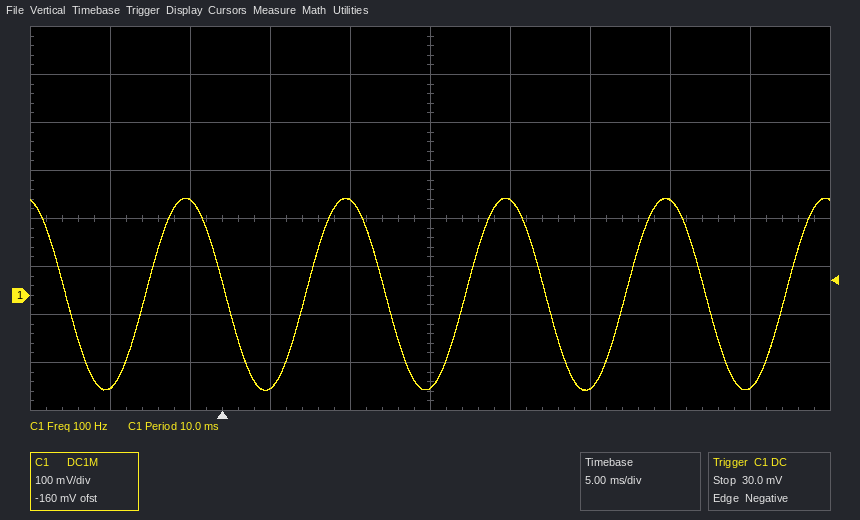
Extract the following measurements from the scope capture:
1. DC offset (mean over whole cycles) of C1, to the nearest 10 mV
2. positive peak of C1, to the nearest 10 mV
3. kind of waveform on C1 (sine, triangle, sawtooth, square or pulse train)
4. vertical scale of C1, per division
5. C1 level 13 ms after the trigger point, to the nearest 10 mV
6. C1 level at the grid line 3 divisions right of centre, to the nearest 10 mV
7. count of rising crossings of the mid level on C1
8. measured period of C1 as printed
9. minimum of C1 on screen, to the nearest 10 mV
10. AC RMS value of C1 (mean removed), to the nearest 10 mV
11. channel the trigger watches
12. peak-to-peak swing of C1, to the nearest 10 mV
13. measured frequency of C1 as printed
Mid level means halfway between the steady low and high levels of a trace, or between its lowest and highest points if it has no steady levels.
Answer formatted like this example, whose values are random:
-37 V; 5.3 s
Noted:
0 mV; 200 mV; sine; 100 mV; -190 mV; 200 mV; 5; 10.0 ms; -200 mV; 140 mV; C1; 400 mV; 100 Hz
